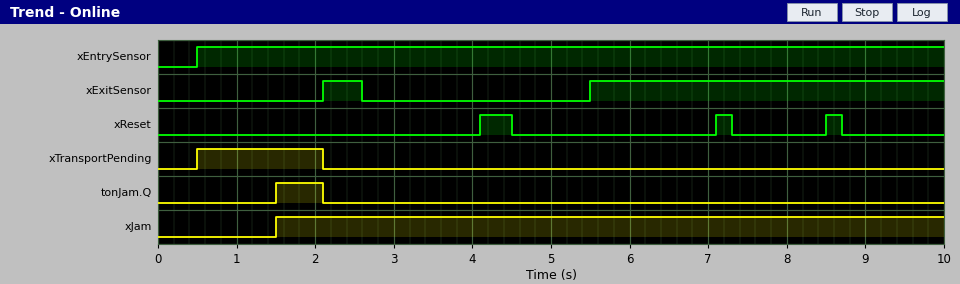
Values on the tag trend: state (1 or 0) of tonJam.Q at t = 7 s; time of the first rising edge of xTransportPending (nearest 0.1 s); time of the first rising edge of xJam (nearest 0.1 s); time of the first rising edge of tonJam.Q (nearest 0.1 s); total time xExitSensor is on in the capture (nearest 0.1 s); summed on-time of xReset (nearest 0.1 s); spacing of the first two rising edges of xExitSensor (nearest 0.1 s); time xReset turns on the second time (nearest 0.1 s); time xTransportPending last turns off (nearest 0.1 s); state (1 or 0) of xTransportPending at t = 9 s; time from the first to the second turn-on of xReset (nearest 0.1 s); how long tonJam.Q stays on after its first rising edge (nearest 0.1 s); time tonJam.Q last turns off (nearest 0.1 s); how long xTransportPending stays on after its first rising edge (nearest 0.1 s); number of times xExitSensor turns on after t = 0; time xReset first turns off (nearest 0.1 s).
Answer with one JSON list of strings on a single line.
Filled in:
["0", "0.5 s", "1.5 s", "1.5 s", "5.0 s", "0.8 s", "3.4 s", "7.1 s", "2.1 s", "0", "3.0 s", "0.6 s", "2.1 s", "1.6 s", "2", "4.5 s"]
